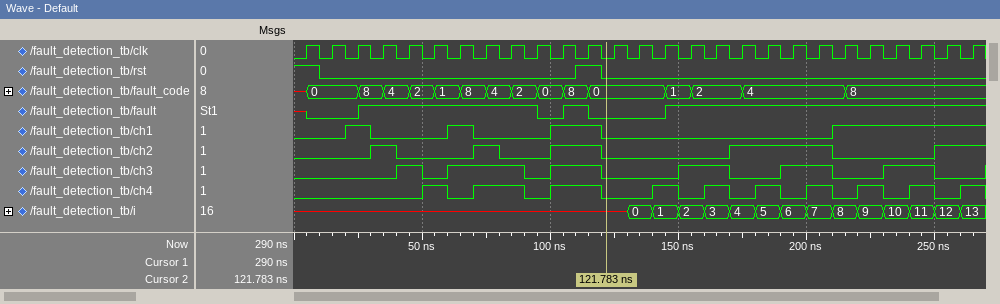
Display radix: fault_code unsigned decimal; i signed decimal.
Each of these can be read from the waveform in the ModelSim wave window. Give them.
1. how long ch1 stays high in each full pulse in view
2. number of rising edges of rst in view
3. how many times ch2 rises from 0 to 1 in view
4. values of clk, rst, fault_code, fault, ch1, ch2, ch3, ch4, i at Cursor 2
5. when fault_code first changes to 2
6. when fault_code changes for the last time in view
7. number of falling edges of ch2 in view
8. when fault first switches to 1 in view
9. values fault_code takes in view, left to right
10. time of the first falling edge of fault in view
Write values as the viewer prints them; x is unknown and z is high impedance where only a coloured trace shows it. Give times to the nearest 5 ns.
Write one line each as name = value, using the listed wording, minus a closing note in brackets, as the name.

how long ch1 stays high in each full pulse in view = 10 ns, 10 ns, 20 ns
number of rising edges of rst in view = 1
how many times ch2 rises from 0 to 1 in view = 5
values of clk, rst, fault_code, fault, ch1, ch2, ch3, ch4, i at Cursor 2 = clk=0, rst=0, fault_code=0, fault=0, ch1=0, ch2=0, ch3=0, ch4=0, i=x
when fault_code first changes to 2 = 45 ns
when fault_code changes for the last time in view = 215 ns
number of falling edges of ch2 in view = 4
when fault first switches to 1 in view = 25 ns
values fault_code takes in view, left to right = x, 0, 8, 4, 2, 1, 8, 4, 2, 0, 8, 0, 1, 2, 4, 8
time of the first falling edge of fault in view = 95 ns
